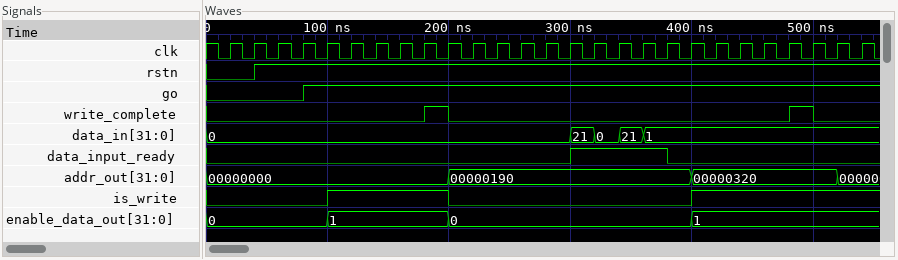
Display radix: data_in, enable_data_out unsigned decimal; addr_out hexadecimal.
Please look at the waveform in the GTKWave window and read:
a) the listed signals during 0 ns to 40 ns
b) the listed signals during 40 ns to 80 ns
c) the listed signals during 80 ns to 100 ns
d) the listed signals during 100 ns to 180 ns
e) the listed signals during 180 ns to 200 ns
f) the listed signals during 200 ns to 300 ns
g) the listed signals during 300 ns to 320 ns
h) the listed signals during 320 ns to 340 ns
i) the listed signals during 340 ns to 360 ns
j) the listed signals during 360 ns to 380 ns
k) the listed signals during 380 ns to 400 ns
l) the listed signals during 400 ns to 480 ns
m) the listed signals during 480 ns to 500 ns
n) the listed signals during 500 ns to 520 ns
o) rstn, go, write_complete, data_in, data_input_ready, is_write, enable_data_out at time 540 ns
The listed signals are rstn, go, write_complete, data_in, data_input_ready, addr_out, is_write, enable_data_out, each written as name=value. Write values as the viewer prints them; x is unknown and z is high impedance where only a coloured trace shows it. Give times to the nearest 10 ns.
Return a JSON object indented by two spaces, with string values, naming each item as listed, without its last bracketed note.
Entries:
{
  "the listed signals during 0 ns to 40 ns": "rstn=0, go=0, write_complete=0, data_in=0, data_input_ready=0, addr_out=00000000, is_write=0, enable_data_out=0",
  "the listed signals during 40 ns to 80 ns": "rstn=1, go=0, write_complete=0, data_in=0, data_input_ready=0, addr_out=00000000, is_write=0, enable_data_out=0",
  "the listed signals during 80 ns to 100 ns": "rstn=1, go=1, write_complete=0, data_in=0, data_input_ready=0, addr_out=00000000, is_write=0, enable_data_out=0",
  "the listed signals during 100 ns to 180 ns": "rstn=1, go=1, write_complete=0, data_in=0, data_input_ready=0, addr_out=00000000, is_write=1, enable_data_out=1",
  "the listed signals during 180 ns to 200 ns": "rstn=1, go=1, write_complete=1, data_in=0, data_input_ready=0, addr_out=00000000, is_write=1, enable_data_out=1",
  "the listed signals during 200 ns to 300 ns": "rstn=1, go=1, write_complete=0, data_in=0, data_input_ready=0, addr_out=00000190, is_write=0, enable_data_out=0",
  "the listed signals during 300 ns to 320 ns": "rstn=1, go=1, write_complete=0, data_in=21, data_input_ready=1, addr_out=00000190, is_write=0, enable_data_out=0",
  "the listed signals during 320 ns to 340 ns": "rstn=1, go=1, write_complete=0, data_in=0, data_input_ready=1, addr_out=00000190, is_write=0, enable_data_out=0",
  "the listed signals during 340 ns to 360 ns": "rstn=1, go=1, write_complete=0, data_in=21, data_input_ready=1, addr_out=00000190, is_write=0, enable_data_out=0",
  "the listed signals during 360 ns to 380 ns": "rstn=1, go=1, write_complete=0, data_in=1, data_input_ready=1, addr_out=00000190, is_write=0, enable_data_out=0",
  "the listed signals during 380 ns to 400 ns": "rstn=1, go=1, write_complete=0, data_in=1, data_input_ready=0, addr_out=00000190, is_write=0, enable_data_out=0",
  "the listed signals during 400 ns to 480 ns": "rstn=1, go=1, write_complete=0, data_in=1, data_input_ready=0, addr_out=00000320, is_write=1, enable_data_out=1",
  "the listed signals during 480 ns to 500 ns": "rstn=1, go=1, write_complete=1, data_in=1, data_input_ready=0, addr_out=00000320, is_write=1, enable_data_out=1",
  "the listed signals during 500 ns to 520 ns": "rstn=1, go=1, write_complete=0, data_in=1, data_input_ready=0, addr_out=00000320, is_write=1, enable_data_out=1",
  "rstn, go, write_complete, data_in, data_input_ready, is_write, enable_data_out at time 540 ns": "rstn=1, go=1, write_complete=0, data_in=1, data_input_ready=0, is_write=1, enable_data_out=1"
}
